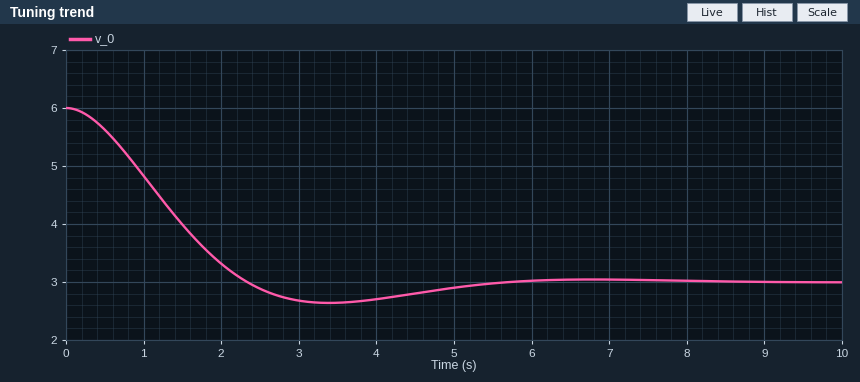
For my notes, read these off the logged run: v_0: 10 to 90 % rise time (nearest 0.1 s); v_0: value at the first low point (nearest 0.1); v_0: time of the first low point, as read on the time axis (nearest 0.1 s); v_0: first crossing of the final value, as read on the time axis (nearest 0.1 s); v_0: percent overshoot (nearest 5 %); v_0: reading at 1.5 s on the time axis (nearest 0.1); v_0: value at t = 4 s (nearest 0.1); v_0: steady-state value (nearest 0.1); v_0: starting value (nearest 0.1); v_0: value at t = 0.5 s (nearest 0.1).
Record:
1.6 s
2.6
3.4 s
2.3 s
10 %
4.0
2.7
3.0
6.0
5.6
